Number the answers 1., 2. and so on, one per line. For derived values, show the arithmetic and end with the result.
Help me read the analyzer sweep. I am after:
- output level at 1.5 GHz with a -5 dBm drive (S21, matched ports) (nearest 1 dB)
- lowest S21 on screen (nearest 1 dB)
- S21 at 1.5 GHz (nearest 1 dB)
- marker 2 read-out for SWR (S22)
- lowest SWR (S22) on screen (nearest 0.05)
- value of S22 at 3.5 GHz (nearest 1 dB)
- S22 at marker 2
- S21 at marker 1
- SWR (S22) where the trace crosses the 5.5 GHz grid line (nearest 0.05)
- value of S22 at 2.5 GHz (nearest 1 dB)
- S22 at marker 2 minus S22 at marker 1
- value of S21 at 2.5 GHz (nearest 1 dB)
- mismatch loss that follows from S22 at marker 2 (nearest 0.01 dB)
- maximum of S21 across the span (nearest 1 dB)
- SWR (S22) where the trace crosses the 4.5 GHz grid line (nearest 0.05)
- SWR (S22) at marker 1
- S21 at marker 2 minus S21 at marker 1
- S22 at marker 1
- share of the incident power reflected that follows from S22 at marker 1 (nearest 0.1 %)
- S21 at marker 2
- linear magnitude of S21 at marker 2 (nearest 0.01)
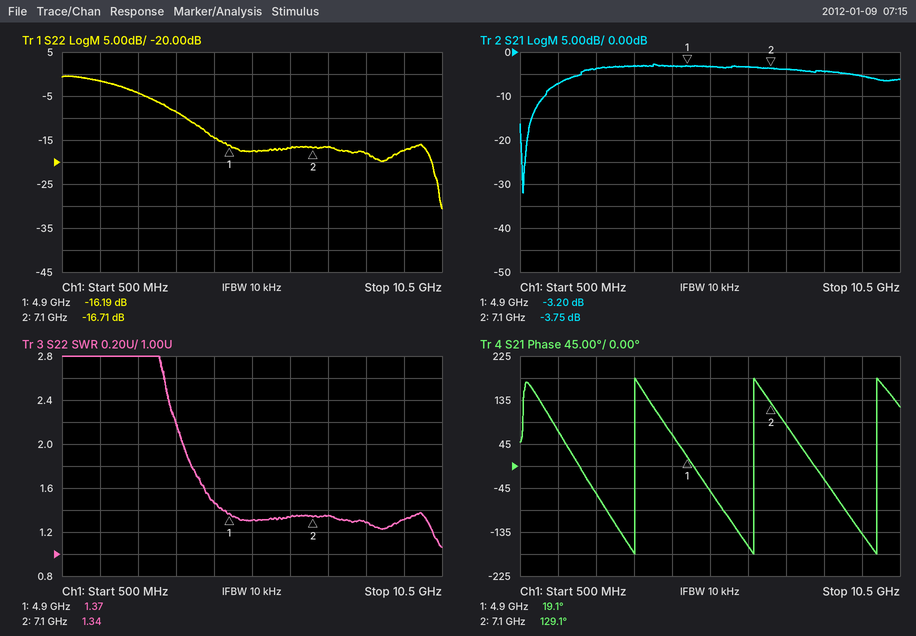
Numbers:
1. -5 dBm + (-7 dB) = -12 dBm
2. -32 dB
3. -7 dB
4. 1.34
5. 1.05
6. -9 dB
7. -16.71 dB
8. -3.20 dB
9. 1.30
10. -4 dB
11. -16.71 − (-16.19) = -0.52 dB
12. -4 dB
13. −10 log10(1 − 10^(-16.71/10)) ≈ 0.09 dB
14. -3 dB
15. 1.45
16. 1.37
17. -3.75 − (-3.2) = -0.55 dB
18. -16.19 dB
19. 10^(-16.19/10) ≈ 2.4 %
20. -3.75 dB
21. 10^(-3.75/20) ≈ 0.65
